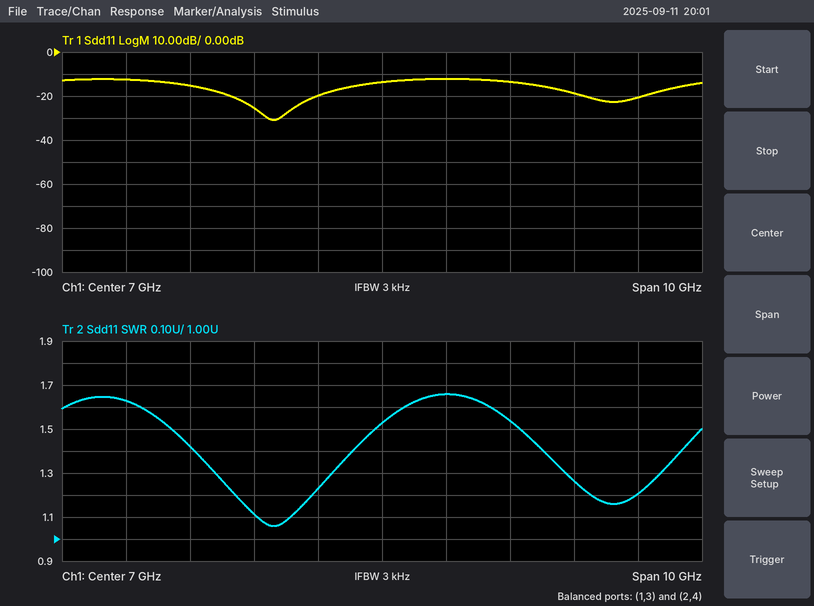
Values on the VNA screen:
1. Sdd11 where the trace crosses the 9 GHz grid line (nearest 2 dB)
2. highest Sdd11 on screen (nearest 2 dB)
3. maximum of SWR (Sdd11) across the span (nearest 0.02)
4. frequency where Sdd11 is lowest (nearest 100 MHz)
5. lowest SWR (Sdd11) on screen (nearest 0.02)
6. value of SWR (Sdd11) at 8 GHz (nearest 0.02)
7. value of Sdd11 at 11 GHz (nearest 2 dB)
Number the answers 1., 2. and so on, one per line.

1. -14 dB
2. -12 dB
3. 1.66
4. 5.3 GHz
5. 1.06
6. 1.66
7. -20 dB
